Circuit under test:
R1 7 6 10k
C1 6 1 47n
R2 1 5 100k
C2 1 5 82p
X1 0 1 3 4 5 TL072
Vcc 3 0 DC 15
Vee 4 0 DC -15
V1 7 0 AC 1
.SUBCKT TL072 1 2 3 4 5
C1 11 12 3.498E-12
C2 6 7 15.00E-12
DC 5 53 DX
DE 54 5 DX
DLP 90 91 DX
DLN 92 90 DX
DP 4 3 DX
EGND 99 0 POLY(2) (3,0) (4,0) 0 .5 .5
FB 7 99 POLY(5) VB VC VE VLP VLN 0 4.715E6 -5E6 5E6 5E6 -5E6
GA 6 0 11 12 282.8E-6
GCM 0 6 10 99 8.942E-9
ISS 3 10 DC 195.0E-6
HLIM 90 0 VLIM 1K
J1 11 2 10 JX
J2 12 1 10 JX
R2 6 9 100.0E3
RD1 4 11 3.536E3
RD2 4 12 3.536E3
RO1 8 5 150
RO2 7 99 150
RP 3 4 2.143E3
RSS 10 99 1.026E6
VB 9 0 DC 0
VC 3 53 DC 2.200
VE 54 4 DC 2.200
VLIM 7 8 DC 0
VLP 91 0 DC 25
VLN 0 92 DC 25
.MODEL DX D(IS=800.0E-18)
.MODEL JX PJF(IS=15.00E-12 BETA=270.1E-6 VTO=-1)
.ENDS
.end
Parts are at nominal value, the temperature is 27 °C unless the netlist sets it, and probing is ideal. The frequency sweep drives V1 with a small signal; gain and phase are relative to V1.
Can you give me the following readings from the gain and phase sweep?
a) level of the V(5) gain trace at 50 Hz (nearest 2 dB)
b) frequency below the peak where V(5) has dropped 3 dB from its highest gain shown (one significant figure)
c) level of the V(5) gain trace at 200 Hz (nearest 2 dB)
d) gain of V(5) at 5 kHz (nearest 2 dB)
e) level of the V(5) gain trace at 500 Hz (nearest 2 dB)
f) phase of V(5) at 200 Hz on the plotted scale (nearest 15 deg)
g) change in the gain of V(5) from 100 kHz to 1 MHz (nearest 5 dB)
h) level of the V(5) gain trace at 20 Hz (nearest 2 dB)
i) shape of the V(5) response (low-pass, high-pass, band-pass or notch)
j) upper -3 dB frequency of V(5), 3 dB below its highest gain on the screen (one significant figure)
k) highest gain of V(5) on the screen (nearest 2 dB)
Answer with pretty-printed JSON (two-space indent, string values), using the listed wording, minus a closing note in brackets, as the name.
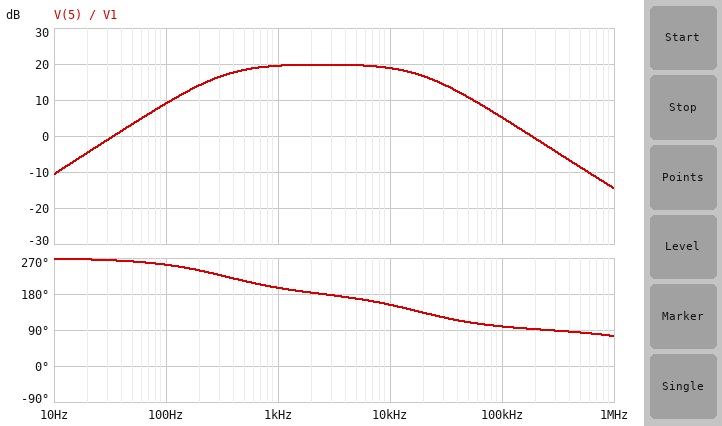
{
  "level of the V(5) gain trace at 50 Hz": "4 dB",
  "frequency below the peak where V(5) has dropped 3 dB from its highest gain shown": "300 Hz",
  "level of the V(5) gain trace at 200 Hz": "14 dB",
  "gain of V(5) at 5 kHz": "20 dB",
  "level of the V(5) gain trace at 500 Hz": "18 dB",
  "phase of V(5) at 200 Hz on the plotted scale": "240 deg",
  "change in the gain of V(5) from 100 kHz to 1 MHz": "-20 dB",
  "level of the V(5) gain trace at 20 Hz": "-4 dB",
  "shape of the V(5) response": "band-pass",
  "upper -3 dB frequency of V(5), 3 dB below its highest gain on the screen": "20 kHz",
  "highest gain of V(5) on the screen": "20 dB"
}
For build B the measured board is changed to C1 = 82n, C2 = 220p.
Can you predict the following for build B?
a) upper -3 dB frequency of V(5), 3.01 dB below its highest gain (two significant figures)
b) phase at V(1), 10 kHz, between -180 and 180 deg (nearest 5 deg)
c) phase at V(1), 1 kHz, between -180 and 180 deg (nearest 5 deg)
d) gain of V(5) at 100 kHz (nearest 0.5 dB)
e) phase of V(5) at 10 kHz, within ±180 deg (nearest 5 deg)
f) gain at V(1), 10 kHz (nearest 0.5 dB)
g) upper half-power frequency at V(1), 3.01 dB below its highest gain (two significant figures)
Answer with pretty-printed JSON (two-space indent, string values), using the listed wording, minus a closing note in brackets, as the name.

{
  "upper -3 dB frequency of V(5), 3.01 dB below its highest gain": "7.5 kHz",
  "phase at V(1), 10 kHz, between -180 and 180 deg": "35 deg",
  "phase at V(1), 1 kHz, between -180 and 180 deg": "90 deg",
  "gain of V(5) at 100 kHz": "-3.0 dB",
  "phase of V(5) at 10 kHz, within ±180 deg": "125 deg",
  "gain at V(1), 10 kHz": "-35.5 dB",
  "upper half-power frequency at V(1), 3.01 dB below its highest gain": "11 MHz"
}
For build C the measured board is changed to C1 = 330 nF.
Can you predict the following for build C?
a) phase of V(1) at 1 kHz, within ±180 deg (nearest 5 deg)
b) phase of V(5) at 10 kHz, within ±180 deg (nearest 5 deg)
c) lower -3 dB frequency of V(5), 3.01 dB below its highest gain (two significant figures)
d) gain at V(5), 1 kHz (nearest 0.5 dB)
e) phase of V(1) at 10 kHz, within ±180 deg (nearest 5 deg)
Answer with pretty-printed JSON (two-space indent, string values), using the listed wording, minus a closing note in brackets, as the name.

{
  "phase of V(1) at 1 kHz, within ±180 deg": "90 deg",
  "phase of V(5) at 10 kHz, within ±180 deg": "150 deg",
  "lower -3 dB frequency of V(5), 3.01 dB below its highest gain": "48 Hz",
  "gain at V(5), 1 kHz": "20.0 dB",
  "phase of V(1) at 10 kHz, within ±180 deg": "60 deg"
}
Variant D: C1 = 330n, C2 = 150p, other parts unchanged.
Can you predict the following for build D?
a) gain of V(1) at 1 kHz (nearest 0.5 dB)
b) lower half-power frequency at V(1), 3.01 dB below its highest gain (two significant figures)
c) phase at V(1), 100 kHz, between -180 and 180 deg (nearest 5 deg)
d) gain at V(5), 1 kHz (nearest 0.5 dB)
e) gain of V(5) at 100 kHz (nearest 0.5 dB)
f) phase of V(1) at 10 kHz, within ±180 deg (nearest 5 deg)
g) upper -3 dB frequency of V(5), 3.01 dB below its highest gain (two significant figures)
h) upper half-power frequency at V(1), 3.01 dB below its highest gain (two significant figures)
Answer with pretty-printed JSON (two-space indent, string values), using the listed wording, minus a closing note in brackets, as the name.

{
  "gain of V(1) at 1 kHz": "-51.0 dB",
  "lower half-power frequency at V(1), 3.01 dB below its highest gain": "14 kHz",
  "phase at V(1), 100 kHz, between -180 and 180 deg": "5 deg",
  "gain at V(5), 1 kHz": "20.0 dB",
  "gain of V(5) at 100 kHz": "0 dB",
  "phase of V(1) at 10 kHz, within ±180 deg": "45 deg",
  "upper -3 dB frequency of V(5), 3.01 dB below its highest gain": "10 kHz",
  "upper half-power frequency at V(1), 3.01 dB below its highest gain": "8.1 MHz"
}
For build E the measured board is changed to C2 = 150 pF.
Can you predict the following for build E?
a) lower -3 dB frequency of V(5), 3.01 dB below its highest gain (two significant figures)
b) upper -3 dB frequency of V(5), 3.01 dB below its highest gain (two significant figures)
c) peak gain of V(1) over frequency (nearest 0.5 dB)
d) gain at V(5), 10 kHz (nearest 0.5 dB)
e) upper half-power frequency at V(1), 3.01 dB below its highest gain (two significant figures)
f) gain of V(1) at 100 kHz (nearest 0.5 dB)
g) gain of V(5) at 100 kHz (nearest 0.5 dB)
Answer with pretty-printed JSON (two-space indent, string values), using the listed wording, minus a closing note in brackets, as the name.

{
  "lower -3 dB frequency of V(5), 3.01 dB below its highest gain": "320 Hz",
  "upper -3 dB frequency of V(5), 3.01 dB below its highest gain": "11 kHz",
  "peak gain of V(1) over frequency": "-29.5 dB",
  "gain at V(5), 10 kHz": "17.0 dB",
  "upper half-power frequency at V(1), 3.01 dB below its highest gain": "8.1 MHz",
  "gain of V(1) at 100 kHz": "-30.5 dB",
  "gain of V(5) at 100 kHz": "0 dB"
}
